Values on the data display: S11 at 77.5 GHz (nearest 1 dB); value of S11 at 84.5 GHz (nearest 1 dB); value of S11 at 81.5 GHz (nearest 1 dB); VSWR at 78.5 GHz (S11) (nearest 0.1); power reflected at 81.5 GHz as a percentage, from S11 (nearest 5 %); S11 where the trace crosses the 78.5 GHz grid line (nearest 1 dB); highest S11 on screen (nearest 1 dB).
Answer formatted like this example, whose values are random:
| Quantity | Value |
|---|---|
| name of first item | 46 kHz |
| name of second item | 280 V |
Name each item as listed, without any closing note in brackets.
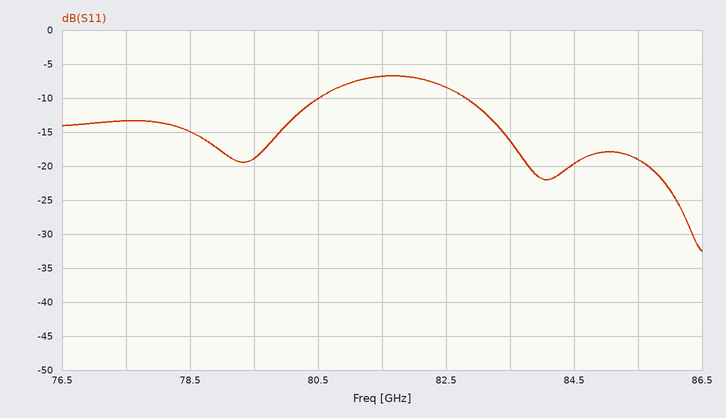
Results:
| Quantity | Value |
|---|---|
| S11 at 77.5 GHz | -13 dB |
| value of S11 at 84.5 GHz | -20 dB |
| value of S11 at 81.5 GHz | -7 dB |
| VSWR at 78.5 GHz (S11) | 1.4 |
| power reflected at 81.5 GHz as a percentage, from S11 | 20 % |
| S11 where the trace crosses the 78.5 GHz grid line | -15 dB |
| highest S11 on screen | -7 dB |
